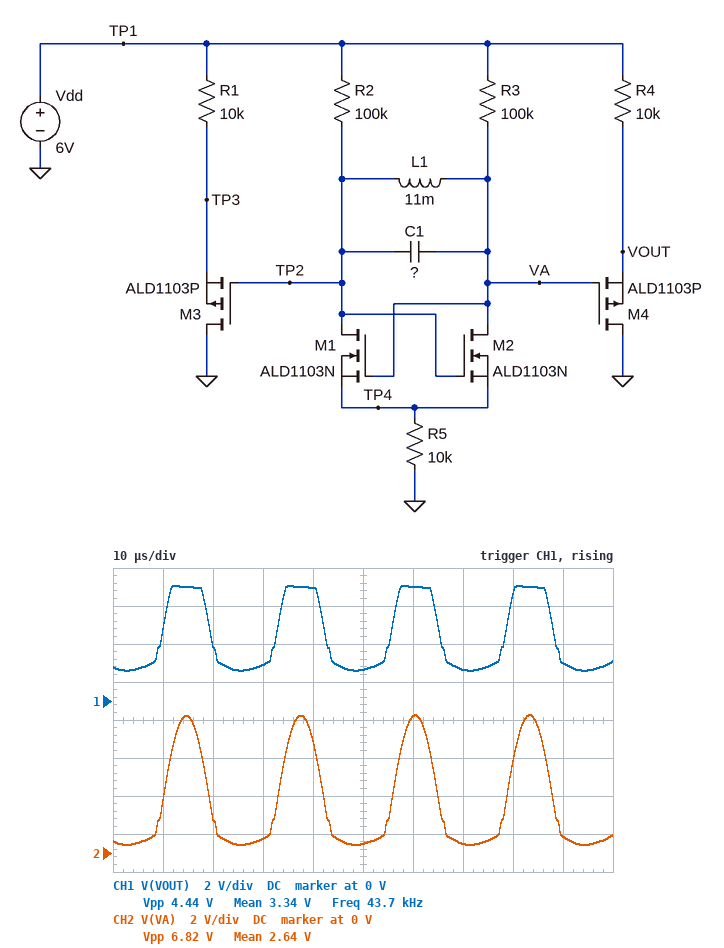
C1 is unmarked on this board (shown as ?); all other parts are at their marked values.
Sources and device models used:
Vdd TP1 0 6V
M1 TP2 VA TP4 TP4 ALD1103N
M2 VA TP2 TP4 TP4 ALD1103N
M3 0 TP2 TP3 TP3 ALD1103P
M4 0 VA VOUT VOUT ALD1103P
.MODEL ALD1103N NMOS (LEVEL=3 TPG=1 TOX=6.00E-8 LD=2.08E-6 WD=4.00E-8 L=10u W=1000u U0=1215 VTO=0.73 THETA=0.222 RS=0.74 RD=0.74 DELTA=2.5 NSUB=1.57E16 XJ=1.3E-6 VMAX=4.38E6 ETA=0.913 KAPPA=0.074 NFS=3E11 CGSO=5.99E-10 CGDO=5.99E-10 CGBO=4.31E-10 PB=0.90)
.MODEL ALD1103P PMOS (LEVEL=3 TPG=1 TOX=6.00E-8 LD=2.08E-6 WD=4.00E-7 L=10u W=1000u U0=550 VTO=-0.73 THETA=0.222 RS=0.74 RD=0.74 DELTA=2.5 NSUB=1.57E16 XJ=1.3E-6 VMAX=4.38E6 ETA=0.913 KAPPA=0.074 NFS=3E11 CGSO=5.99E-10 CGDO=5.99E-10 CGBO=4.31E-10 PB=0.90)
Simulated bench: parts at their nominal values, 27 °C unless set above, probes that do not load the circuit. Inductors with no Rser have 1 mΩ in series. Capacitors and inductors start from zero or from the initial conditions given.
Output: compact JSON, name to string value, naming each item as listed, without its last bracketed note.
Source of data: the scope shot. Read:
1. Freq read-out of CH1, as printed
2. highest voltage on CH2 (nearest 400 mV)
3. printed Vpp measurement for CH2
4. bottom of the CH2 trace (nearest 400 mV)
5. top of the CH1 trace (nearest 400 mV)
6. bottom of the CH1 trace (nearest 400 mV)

{"Freq read-out of CH1, as printed": "43.7 kHz", "highest voltage on CH2": "7.2 V", "printed Vpp measurement for CH2": "6.82 V", "bottom of the CH2 trace": "400 mV", "top of the CH1 trace": "6.0 V", "bottom of the CH1 trace": "1.6 V"}
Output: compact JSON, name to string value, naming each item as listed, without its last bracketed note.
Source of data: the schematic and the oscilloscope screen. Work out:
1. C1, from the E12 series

{"C1, from the E12 series": "1.2 nF"}
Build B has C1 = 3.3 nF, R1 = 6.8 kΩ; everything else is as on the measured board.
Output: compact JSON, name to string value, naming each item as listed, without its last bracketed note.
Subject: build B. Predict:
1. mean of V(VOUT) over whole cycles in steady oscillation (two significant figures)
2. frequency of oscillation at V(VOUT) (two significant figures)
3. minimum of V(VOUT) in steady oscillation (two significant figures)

{"mean of V(VOUT) over whole cycles in steady oscillation": "3.4 V", "frequency of oscillation at V(VOUT)": "26 kHz", "minimum of V(VOUT) in steady oscillation": "1.7 V"}
